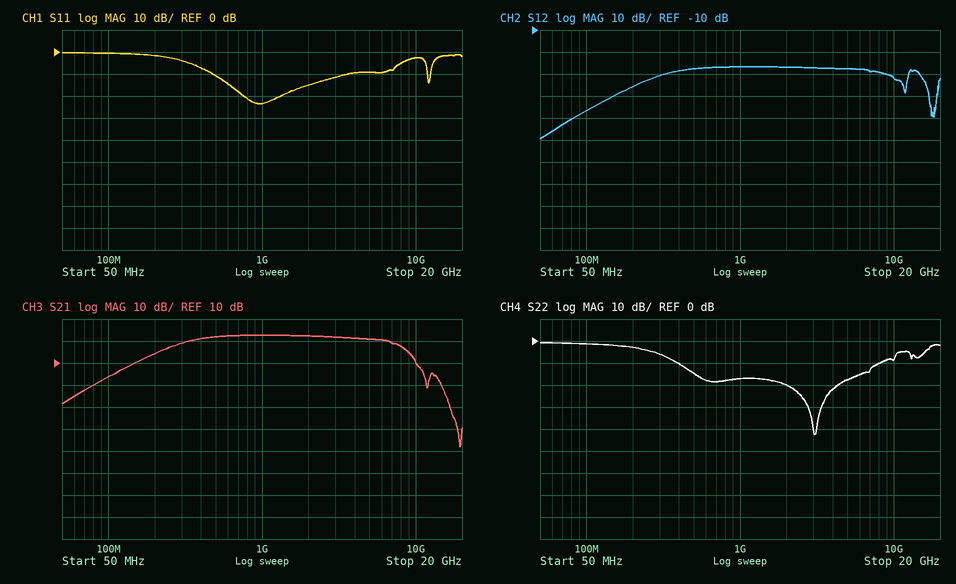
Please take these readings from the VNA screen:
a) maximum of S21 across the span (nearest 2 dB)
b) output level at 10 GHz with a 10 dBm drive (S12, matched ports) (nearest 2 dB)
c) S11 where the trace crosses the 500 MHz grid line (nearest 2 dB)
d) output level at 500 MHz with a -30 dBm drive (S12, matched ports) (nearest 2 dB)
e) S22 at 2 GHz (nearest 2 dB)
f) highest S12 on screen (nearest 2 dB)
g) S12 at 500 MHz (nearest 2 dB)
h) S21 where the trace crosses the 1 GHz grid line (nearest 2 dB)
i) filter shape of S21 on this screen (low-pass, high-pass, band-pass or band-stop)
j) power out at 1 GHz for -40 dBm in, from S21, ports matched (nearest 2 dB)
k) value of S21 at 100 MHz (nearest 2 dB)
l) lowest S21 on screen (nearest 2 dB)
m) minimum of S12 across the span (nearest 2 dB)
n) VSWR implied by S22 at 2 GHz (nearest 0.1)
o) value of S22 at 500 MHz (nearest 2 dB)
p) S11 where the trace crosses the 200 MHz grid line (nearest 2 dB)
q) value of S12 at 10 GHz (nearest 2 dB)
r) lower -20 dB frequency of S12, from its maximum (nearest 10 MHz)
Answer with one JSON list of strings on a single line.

["22 dB", "-22 dBm", "-10 dB", "-58 dBm", "-20 dB", "-26 dB", "-28 dB", "22 dB", "band-pass", "-18 dBm", "4 dB", "-28 dB", "-60 dB", "1.2", "-14 dB", "-2 dB", "-32 dB", "100 MHz"]
